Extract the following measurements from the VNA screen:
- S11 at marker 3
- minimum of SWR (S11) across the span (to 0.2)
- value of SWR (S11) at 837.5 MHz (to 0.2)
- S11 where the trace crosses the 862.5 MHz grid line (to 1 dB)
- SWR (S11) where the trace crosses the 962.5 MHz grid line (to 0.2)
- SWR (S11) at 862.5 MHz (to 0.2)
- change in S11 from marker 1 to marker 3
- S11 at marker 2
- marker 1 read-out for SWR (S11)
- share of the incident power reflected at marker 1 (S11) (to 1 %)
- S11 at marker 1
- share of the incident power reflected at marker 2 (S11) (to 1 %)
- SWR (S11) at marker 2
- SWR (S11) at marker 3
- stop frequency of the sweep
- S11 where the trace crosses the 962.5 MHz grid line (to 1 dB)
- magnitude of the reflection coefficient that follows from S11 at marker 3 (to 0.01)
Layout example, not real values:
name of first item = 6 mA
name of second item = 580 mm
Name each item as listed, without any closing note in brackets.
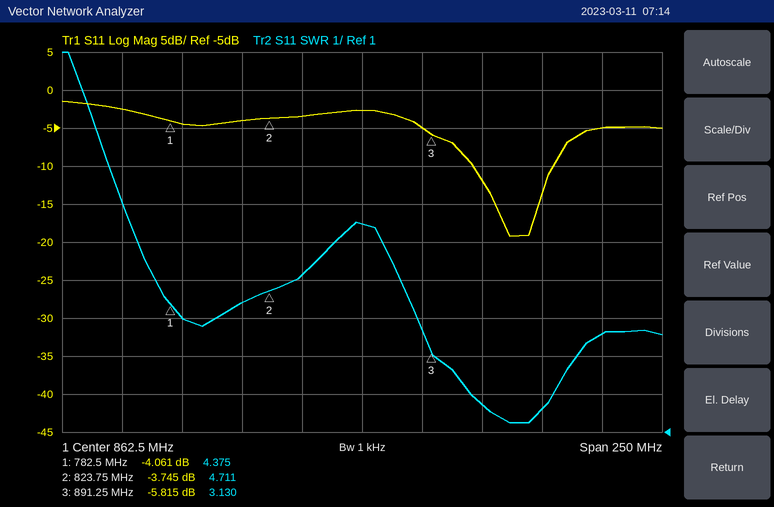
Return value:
S11 at marker 3 = -5.815 dB
minimum of SWR (S11) across the span = 1.2
value of SWR (S11) at 837.5 MHz = 5.2
S11 where the trace crosses the 862.5 MHz grid line = -3 dB
SWR (S11) where the trace crosses the 962.5 MHz grid line = 3.6
SWR (S11) at 862.5 MHz = 6.4
change in S11 from marker 1 to marker 3 = -1.754 dB
S11 at marker 2 = -3.745 dB
marker 1 read-out for SWR = 4.375
share of the incident power reflected at marker 1 (S11) = 39 %
S11 at marker 1 = -4.061 dB
share of the incident power reflected at marker 2 (S11) = 42 %
SWR (S11) at marker 2 = 4.711
SWR (S11) at marker 3 = 3.130
stop frequency of the sweep = 987.5 MHz
S11 where the trace crosses the 962.5 MHz grid line = -5 dB
magnitude of the reflection coefficient that follows from S11 at marker 3 = 0.51
